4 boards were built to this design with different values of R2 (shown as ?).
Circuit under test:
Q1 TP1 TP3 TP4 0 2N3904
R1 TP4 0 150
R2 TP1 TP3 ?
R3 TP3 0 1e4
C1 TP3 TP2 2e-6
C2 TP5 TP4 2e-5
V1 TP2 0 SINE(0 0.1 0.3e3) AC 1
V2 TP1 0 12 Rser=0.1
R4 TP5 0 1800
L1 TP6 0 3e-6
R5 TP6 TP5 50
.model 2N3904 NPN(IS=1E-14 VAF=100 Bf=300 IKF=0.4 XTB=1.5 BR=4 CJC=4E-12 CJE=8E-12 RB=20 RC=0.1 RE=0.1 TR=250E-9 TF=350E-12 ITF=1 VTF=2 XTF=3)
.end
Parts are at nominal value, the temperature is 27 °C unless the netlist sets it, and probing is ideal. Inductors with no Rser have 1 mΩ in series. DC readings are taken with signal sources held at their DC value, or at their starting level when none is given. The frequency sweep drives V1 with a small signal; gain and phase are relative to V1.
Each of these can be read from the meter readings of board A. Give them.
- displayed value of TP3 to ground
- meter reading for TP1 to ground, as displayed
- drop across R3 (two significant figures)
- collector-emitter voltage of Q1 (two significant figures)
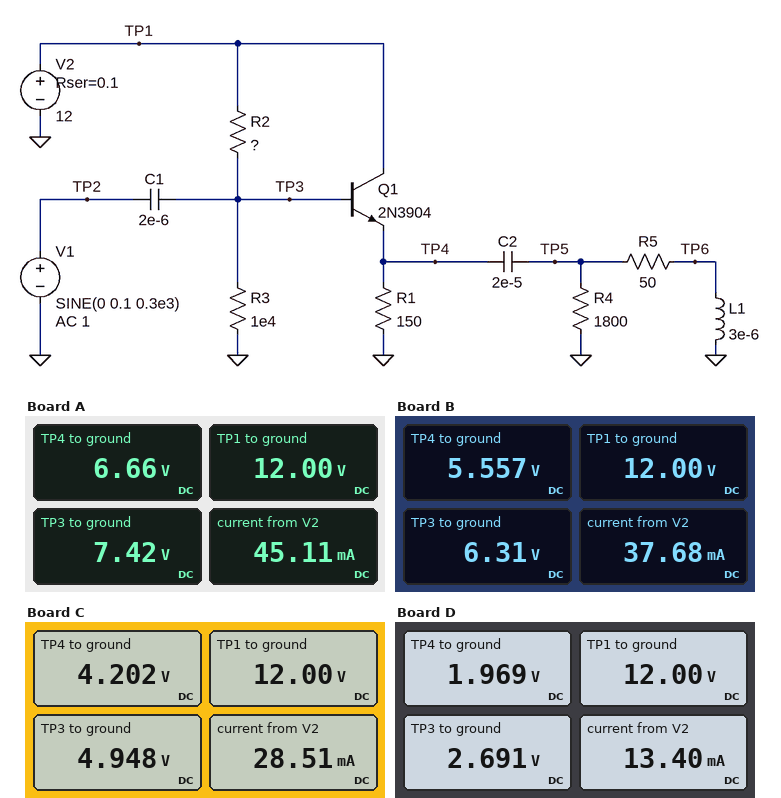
7.42 V
12.00 V
7.4 V
5.3 V
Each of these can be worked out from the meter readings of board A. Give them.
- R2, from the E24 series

5.1 kΩ
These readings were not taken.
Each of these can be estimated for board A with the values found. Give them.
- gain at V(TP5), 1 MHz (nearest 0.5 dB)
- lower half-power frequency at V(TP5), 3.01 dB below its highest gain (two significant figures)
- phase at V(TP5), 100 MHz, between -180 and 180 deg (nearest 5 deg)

0 dB
180 Hz
-5 deg
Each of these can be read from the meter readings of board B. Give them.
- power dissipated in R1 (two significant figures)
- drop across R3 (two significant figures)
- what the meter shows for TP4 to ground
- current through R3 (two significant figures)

210 mW
6.3 V
5.557 V
630 µA
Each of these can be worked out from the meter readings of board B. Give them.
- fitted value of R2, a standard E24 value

7.5 kΩ
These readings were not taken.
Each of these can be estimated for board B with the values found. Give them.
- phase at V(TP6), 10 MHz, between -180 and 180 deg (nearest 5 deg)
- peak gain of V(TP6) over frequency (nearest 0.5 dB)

15 deg
0 dB
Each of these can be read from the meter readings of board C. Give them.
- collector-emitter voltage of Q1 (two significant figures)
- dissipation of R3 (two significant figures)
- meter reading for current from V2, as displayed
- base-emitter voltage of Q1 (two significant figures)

7.8 V
2.4 mW
28.51 mA
750 mV
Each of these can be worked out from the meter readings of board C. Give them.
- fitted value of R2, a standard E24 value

12 kΩ
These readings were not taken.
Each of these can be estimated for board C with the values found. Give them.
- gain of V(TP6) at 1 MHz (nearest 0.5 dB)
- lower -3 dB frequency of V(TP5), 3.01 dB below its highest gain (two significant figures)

-9.5 dB
170 Hz
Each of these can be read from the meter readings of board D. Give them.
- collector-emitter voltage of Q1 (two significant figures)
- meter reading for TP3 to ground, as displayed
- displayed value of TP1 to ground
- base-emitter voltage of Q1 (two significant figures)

10 V
2.691 V
12.00 V
720 mV
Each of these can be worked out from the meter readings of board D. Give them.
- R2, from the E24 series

30 kΩ
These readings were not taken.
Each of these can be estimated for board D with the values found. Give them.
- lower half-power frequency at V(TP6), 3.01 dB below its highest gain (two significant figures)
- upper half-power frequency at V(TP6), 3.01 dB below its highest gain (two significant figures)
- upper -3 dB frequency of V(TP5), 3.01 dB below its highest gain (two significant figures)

2.7 MHz
4.0 GHz
4.0 GHz
